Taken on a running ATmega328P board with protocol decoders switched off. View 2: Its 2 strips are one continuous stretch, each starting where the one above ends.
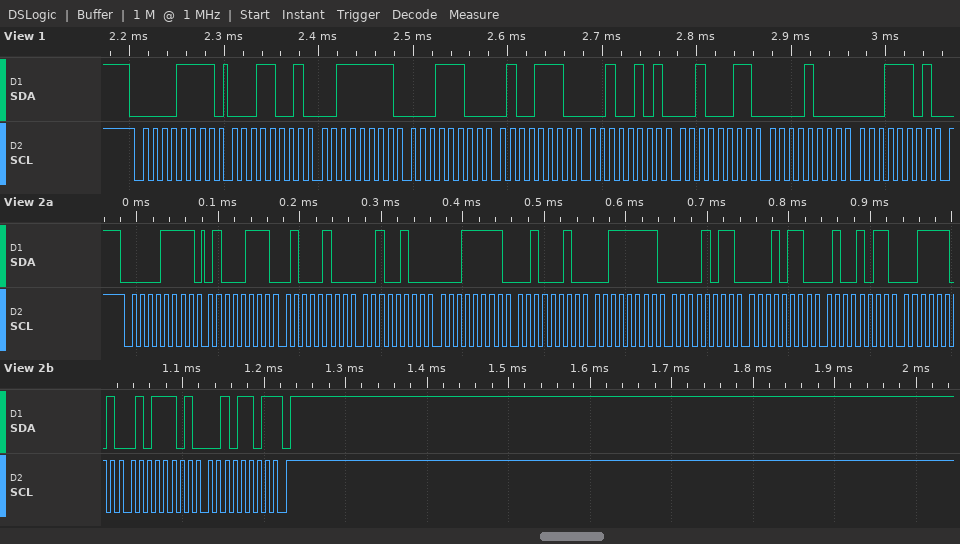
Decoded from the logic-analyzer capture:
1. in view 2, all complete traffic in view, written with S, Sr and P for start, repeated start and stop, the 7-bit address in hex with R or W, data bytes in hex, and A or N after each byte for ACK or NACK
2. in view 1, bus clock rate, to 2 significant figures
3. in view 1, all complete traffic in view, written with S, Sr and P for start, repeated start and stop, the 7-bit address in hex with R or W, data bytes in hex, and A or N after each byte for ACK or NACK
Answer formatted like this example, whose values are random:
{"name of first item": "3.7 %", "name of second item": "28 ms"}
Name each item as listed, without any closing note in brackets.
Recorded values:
{"in view 2, all complete traffic in view, written with S, Sr and P for start, repeated start and stop, the 7-bit address in hex with R or W, data bytes in hex, and A or N after each byte for ACK or NACK": "S 07R A 47 A 44 A 24 A 1F A 22 A 3F A 0B A 16 A 4B A 3D A 5D A 2D N P", "in view 1, bus clock rate, to 2 significant figures": "100 kHz", "in view 1, all complete traffic in view, written with S, Sr and P for start, repeated start and stop, the 7-bit address in hex with R or W, data bytes in hex, and A or N after each byte for ACK or NACK": "S 07R A 19 A 3F A 1C A 4E A 25 A 23 A 08 A 1D A"}
